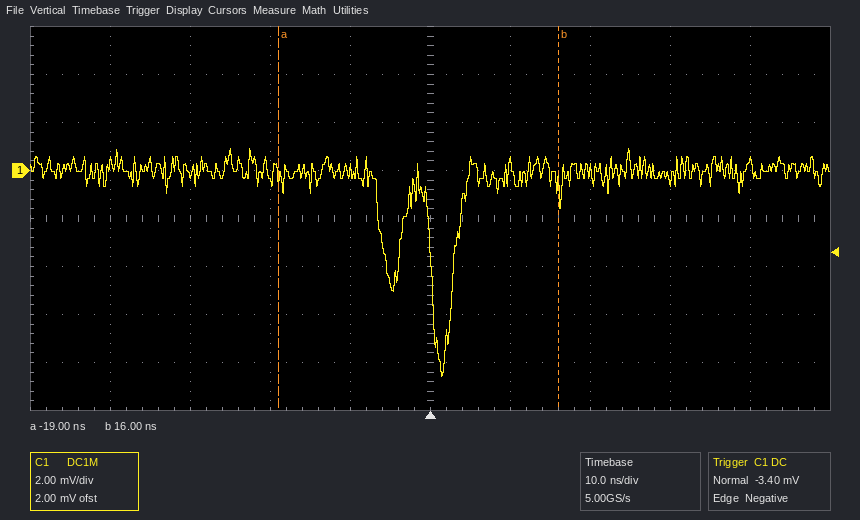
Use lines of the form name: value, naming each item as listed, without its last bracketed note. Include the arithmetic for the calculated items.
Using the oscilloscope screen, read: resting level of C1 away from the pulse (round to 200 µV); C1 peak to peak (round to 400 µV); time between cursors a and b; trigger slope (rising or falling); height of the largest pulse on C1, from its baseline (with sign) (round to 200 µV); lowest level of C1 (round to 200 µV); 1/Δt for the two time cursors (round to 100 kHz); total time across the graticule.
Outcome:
resting level of C1 away from the pulse: 0.0 mV
C1 peak to peak: 9.6 mV
time between cursors a and b: 16 ns − (-19 ns) = 35 ns
trigger slope: falling
height of the largest pulse on C1, from its baseline (with sign): -8.6 mV − (0.0 mV) = -8.6 mV
lowest level of C1: -8.6 mV
1/Δt for the two time cursors: 1 / 35 ns ≈ 28.6 MHz
total time across the graticule: 100 ns
